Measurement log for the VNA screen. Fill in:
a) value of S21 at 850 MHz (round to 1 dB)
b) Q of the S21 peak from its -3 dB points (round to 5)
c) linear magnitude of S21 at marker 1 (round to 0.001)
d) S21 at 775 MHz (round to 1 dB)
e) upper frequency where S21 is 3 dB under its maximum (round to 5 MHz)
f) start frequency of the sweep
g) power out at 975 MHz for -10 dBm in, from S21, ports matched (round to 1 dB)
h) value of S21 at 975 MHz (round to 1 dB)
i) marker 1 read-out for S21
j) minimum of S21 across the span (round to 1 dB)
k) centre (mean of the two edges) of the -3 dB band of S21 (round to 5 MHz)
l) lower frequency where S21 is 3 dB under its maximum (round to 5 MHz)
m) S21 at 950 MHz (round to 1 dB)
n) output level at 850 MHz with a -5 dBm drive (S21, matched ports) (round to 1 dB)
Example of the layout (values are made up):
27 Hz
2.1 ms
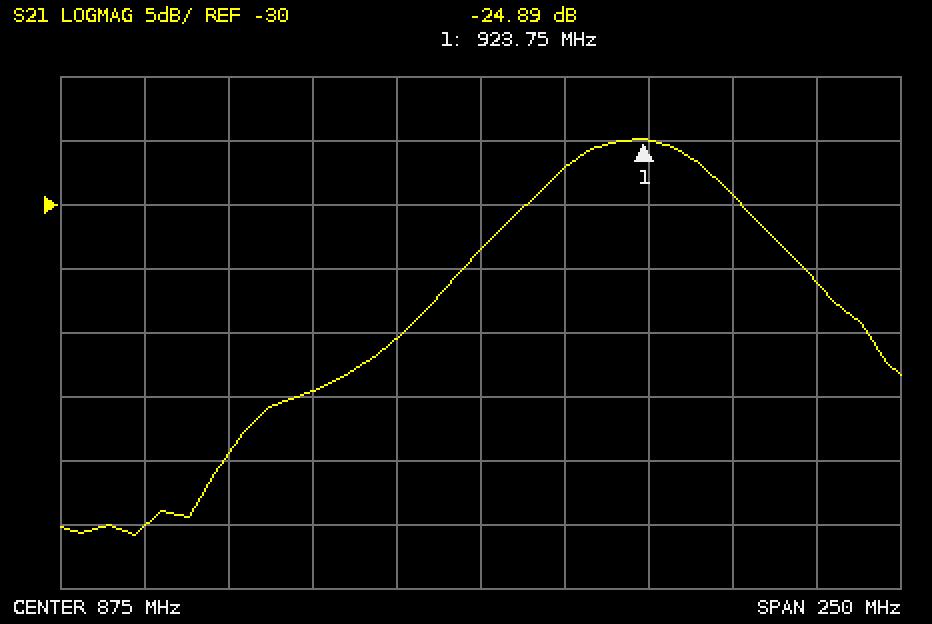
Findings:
-40 dB
20
0.057
-55 dB
945 MHz
750 MHz
-46 dBm
-36 dB
-24.89 dB
-56 dB
920 MHz
895 MHz
-29 dB
-45 dBm
